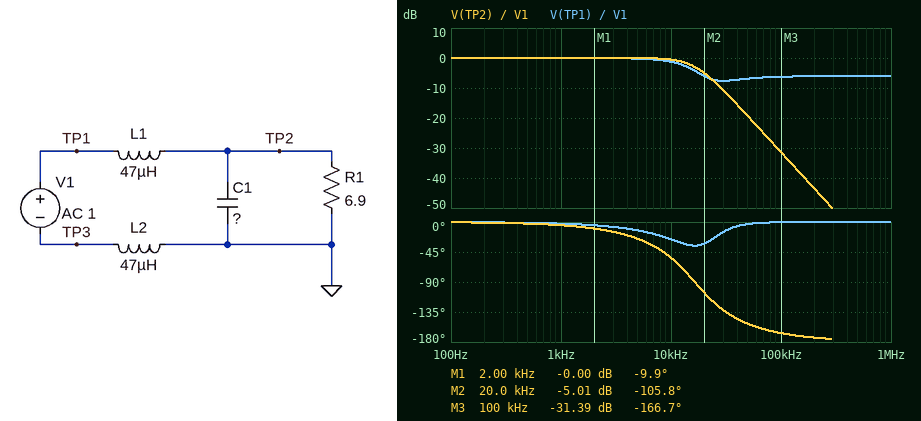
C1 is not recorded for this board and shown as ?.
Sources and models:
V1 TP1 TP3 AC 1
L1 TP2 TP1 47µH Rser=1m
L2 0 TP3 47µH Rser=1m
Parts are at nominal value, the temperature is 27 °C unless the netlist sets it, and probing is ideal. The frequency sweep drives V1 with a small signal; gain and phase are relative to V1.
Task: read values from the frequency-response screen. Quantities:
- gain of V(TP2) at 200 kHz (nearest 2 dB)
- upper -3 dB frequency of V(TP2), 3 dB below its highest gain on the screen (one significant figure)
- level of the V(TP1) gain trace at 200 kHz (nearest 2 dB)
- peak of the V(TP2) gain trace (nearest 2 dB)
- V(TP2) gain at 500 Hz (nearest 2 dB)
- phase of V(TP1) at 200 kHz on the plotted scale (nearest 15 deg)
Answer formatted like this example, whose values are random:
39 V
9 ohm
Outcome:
-44 dB
20 kHz
-6 dB
0 dB
0 dB
0 deg
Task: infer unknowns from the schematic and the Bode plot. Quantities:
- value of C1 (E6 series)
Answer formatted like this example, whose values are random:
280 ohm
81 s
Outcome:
1 µF
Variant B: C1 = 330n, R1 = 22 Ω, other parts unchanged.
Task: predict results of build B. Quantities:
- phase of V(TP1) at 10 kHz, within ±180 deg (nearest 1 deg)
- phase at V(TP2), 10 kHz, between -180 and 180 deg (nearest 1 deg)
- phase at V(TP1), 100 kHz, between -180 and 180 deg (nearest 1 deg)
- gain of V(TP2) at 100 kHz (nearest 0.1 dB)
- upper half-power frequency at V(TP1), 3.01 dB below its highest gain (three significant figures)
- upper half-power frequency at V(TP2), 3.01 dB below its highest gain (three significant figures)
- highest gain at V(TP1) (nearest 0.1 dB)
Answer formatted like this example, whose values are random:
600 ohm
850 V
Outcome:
-9 deg
-17 deg
-1 deg
-21.3 dB
29.6 kHz
34.0 kHz
0.7 dB
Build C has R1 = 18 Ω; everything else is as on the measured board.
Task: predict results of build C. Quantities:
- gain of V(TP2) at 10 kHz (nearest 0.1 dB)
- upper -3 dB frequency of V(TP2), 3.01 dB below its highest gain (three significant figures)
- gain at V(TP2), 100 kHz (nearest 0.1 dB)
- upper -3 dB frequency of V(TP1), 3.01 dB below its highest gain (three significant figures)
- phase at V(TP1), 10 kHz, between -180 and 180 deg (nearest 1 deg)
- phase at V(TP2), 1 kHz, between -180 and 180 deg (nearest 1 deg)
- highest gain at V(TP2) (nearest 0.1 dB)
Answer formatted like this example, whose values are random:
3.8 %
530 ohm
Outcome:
3.0 dB
19.2 kHz
-31.2 dB
17.4 kHz
-16 deg
-2 deg
5.7 dB
